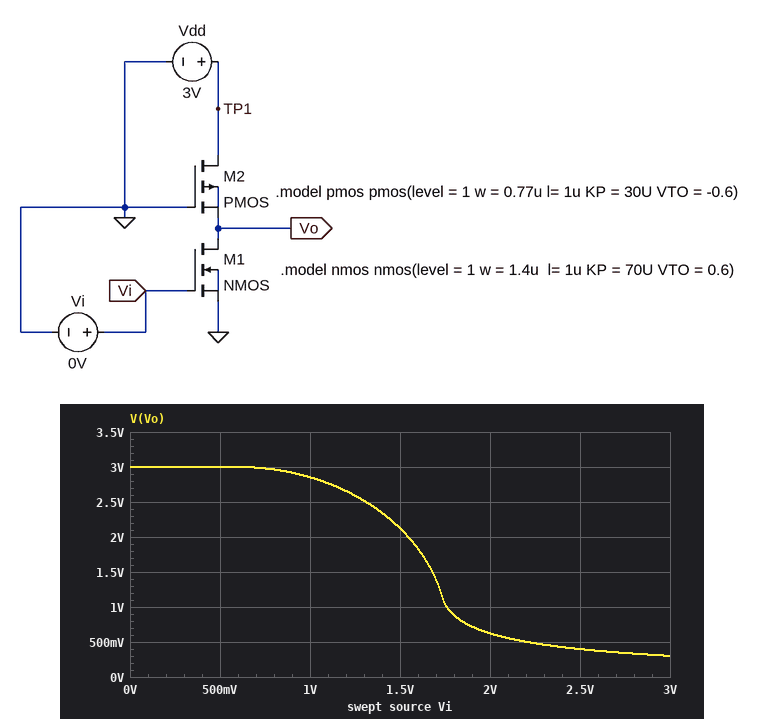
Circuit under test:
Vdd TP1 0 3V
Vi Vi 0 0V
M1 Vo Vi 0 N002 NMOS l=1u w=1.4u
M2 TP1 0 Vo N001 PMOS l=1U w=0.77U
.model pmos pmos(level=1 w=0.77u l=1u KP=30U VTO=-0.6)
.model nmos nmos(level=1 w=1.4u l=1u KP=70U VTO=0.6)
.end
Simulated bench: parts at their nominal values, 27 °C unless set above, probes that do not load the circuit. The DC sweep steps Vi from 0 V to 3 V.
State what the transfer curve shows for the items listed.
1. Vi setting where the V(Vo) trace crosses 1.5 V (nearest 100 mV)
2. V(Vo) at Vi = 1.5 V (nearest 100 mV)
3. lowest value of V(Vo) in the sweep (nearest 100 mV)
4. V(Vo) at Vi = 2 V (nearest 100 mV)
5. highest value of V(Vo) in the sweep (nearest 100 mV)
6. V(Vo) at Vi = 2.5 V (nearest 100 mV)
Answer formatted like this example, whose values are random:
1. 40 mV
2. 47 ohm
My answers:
1. 1.7 V
2. 2.1 V
3. 300 mV
4. 600 mV
5. 3.0 V
6. 400 mV
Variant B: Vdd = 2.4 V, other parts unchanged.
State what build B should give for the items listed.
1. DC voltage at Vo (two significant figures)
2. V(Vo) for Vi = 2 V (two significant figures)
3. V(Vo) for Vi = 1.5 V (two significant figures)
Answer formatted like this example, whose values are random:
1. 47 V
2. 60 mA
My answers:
1. 2.4 V
2. 310 mV
3. 680 mV
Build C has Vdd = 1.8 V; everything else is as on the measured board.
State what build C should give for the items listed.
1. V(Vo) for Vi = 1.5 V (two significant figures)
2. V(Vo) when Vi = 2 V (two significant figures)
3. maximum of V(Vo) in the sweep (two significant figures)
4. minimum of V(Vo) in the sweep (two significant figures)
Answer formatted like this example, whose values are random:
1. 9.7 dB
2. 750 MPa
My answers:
1. 210 mV
2. 130 mV
3. 1.8 V
4. 72 mV
